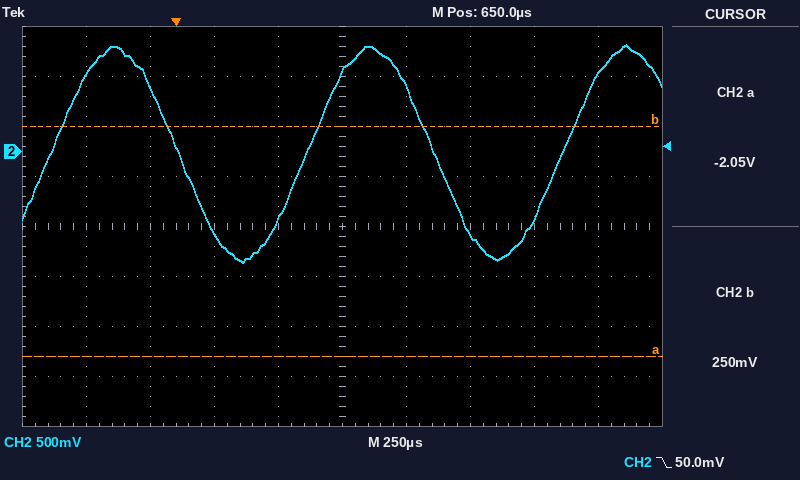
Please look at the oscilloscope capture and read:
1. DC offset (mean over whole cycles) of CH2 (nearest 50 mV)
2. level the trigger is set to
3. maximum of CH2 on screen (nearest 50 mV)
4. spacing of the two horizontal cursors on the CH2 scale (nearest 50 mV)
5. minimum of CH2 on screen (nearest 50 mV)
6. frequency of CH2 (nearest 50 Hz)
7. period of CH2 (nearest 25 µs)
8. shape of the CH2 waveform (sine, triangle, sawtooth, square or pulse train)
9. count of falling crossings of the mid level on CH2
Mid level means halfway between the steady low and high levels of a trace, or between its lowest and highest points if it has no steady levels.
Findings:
0 mV
50.0 mV
1.05 V
2.30 V
-1.10 V
1.00 kHz
1.000 ms
sine
2
